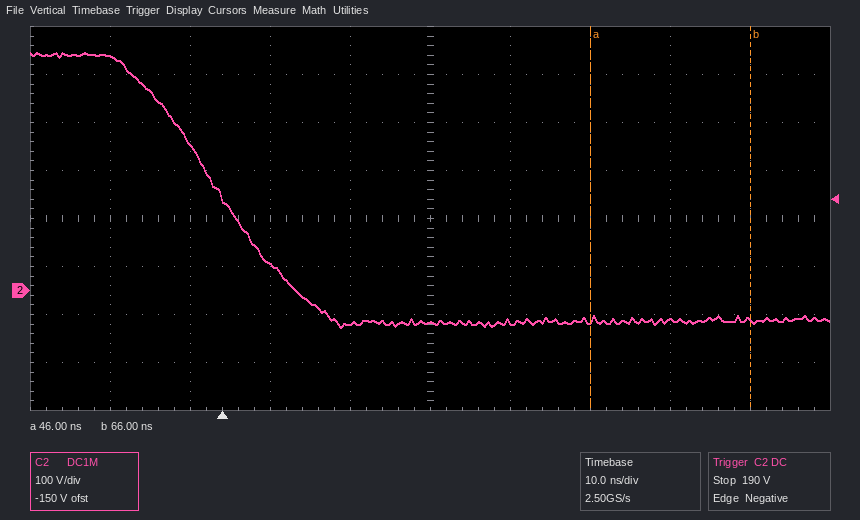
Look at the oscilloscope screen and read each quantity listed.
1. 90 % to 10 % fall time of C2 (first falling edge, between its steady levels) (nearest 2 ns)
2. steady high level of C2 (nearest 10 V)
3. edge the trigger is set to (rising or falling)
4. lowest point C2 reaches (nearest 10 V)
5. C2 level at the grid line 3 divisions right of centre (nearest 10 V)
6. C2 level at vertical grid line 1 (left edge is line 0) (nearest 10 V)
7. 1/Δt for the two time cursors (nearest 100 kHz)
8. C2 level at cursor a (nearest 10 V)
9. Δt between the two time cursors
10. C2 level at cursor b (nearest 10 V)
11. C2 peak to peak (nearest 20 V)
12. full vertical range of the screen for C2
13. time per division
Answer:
20 ns
490 V
falling
-80 V
-60 V
490 V
50.0 MHz
-60 V
20 ns
-60 V
580 V
800 V
10 ns
